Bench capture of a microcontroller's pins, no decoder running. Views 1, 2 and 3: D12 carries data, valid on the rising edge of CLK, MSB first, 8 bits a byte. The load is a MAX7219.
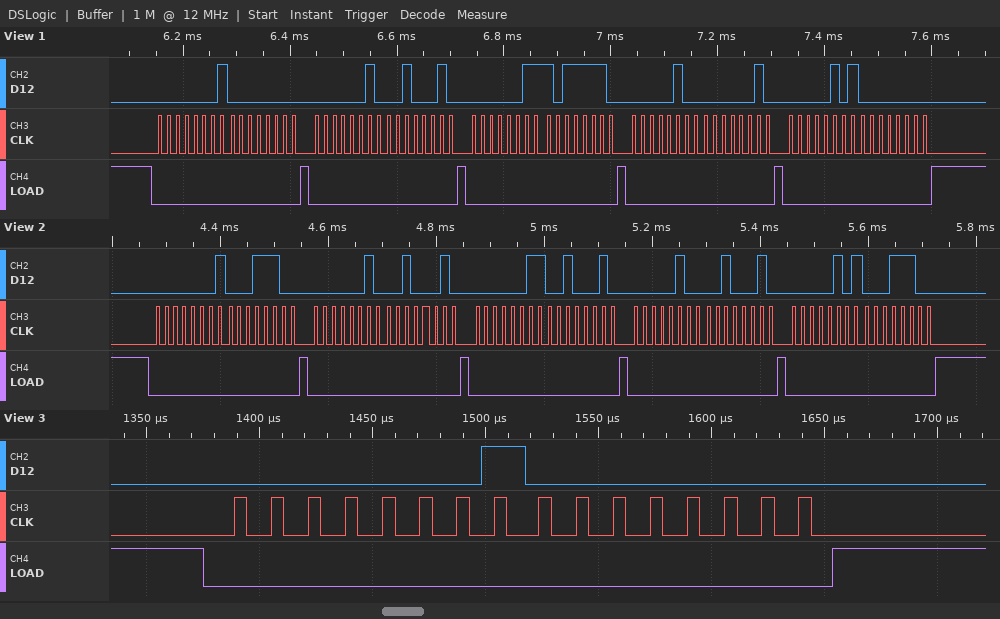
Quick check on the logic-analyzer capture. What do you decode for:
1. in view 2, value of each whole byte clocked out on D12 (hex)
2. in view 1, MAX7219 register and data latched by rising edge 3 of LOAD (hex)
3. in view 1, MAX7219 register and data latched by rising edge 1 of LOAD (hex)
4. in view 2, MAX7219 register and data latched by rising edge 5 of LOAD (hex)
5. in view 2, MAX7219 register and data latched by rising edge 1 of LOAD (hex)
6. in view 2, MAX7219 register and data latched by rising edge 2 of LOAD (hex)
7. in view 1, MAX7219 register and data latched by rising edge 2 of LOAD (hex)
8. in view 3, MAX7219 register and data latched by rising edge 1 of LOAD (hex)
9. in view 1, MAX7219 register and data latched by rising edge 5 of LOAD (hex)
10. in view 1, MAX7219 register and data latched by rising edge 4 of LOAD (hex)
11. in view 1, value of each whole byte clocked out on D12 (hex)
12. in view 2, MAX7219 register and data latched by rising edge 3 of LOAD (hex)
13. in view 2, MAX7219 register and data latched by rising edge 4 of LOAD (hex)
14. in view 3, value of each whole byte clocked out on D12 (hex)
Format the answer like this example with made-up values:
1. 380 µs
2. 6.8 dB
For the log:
1. 01 1C 02 22 03 22 04 22 05 1C
2. register 0x3, data 0xBE
3. register 0x1, data 0x00
4. register 0x5, data 0x1C
5. register 0x1, data 0x1C
6. register 0x2, data 0x22
7. register 0x2, data 0x22
8. register 0x1, data 0x00
9. register 0x5, data 0x00
10. register 0x4, data 0x02
11. 01 00 02 22 03 BE 04 02 05 00
12. register 0x3, data 0x22
13. register 0x4, data 0x22
14. 0x01 0x00
